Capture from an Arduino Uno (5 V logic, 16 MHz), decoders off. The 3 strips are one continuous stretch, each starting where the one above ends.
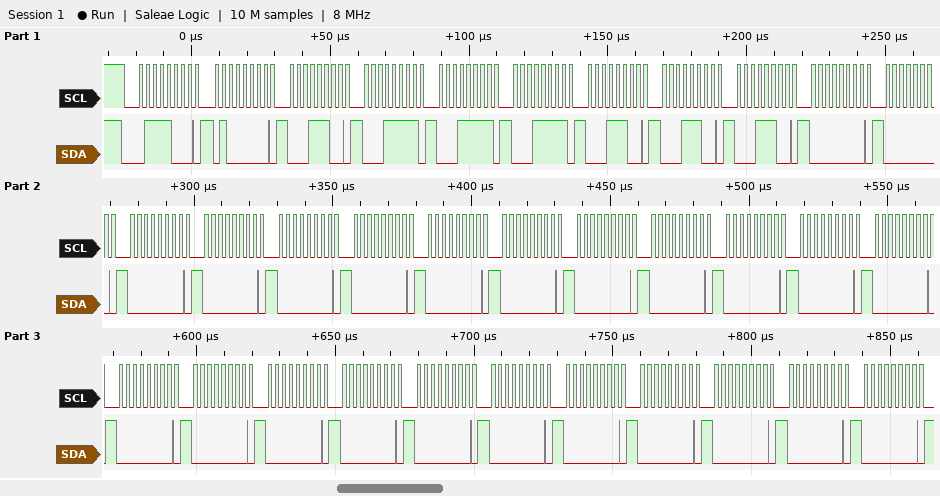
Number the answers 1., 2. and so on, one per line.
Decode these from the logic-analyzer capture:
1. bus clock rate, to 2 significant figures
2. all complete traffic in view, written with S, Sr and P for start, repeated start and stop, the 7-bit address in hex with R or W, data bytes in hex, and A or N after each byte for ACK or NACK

1. 400 kHz
2. S 3CW A 40 A 1C A 1F A 1F A 1F A 1C A 1C A 1C A 00 A 00 A 00 A 00 A 00 A 00 A 00 A 00 A 00 A 00 A 00 A 00 A 00 A 00 A 00 A 00 A 00 A 00 A 00 A 00 A 00 A 00 A 00 A 00 A
